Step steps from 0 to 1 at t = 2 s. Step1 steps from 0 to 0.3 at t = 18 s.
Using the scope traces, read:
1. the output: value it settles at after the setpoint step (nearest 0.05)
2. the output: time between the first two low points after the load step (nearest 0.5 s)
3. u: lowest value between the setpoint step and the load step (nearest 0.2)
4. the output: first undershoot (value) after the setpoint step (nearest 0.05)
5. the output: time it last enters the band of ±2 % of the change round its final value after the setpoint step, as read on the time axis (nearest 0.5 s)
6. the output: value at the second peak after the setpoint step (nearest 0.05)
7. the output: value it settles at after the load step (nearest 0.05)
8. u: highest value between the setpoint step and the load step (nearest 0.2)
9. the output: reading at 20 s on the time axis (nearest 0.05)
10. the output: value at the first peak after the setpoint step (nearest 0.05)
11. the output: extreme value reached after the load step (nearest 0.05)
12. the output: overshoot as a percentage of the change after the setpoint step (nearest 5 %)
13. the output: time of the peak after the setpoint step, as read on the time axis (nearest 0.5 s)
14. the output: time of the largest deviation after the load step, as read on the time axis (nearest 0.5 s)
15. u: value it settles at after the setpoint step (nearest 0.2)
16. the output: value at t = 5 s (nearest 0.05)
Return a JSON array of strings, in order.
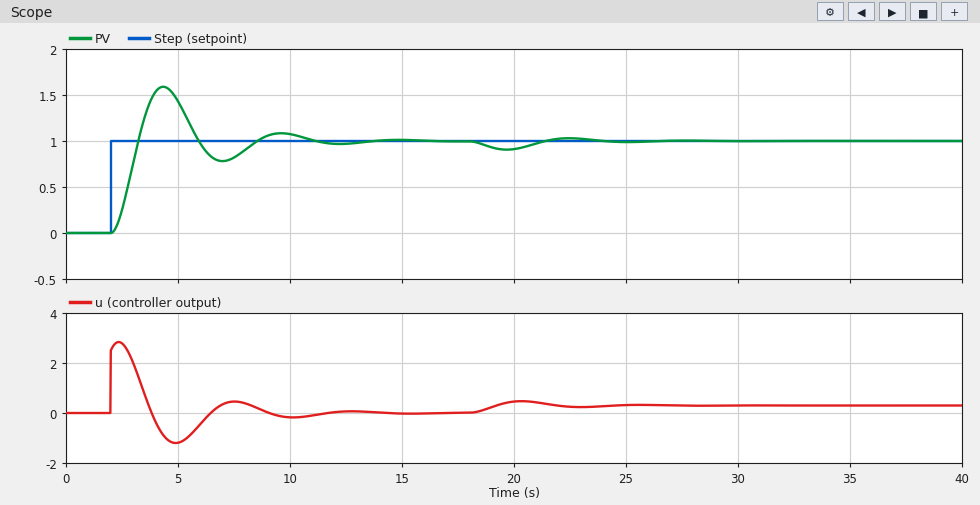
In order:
["1.00", "5.5 s", "-1.2", "0.80", "13.0 s", "1.10", "1.00", "2.8", "0.90", "1.60", "0.90", "60 %", "4.5 s", "19.5 s", "0.0", "1.45"]
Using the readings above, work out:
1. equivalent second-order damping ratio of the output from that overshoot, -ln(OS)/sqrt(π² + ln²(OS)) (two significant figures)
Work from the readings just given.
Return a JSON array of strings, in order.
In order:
["0.16"]
